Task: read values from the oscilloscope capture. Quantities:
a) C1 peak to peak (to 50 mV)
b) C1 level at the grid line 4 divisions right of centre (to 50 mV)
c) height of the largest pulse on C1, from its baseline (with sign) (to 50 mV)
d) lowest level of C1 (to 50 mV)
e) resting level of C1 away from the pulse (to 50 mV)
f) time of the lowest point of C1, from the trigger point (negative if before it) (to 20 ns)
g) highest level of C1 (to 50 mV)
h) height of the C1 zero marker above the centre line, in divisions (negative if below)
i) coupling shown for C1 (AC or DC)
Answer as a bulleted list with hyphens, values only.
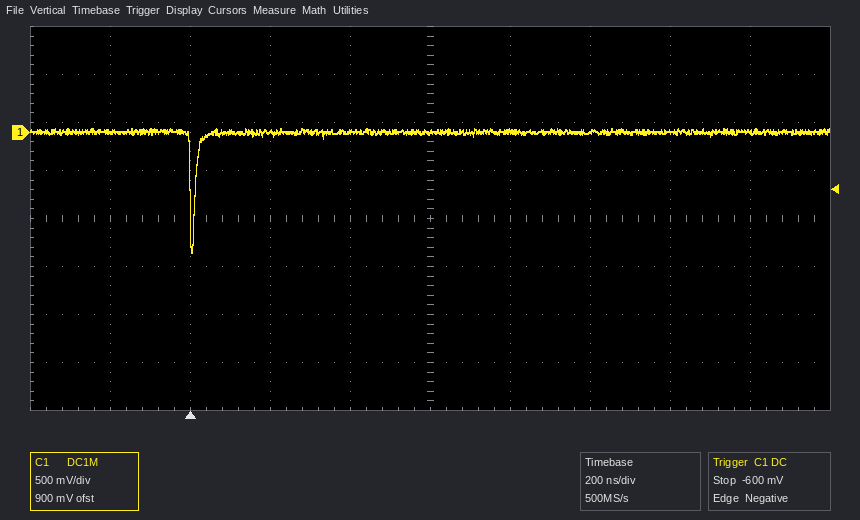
- 1.30 V
- 0 mV
- -1.25 V
- -1.25 V
- 0 mV
- 0 ns
- 50 mV
- +1.8 div
- DC
